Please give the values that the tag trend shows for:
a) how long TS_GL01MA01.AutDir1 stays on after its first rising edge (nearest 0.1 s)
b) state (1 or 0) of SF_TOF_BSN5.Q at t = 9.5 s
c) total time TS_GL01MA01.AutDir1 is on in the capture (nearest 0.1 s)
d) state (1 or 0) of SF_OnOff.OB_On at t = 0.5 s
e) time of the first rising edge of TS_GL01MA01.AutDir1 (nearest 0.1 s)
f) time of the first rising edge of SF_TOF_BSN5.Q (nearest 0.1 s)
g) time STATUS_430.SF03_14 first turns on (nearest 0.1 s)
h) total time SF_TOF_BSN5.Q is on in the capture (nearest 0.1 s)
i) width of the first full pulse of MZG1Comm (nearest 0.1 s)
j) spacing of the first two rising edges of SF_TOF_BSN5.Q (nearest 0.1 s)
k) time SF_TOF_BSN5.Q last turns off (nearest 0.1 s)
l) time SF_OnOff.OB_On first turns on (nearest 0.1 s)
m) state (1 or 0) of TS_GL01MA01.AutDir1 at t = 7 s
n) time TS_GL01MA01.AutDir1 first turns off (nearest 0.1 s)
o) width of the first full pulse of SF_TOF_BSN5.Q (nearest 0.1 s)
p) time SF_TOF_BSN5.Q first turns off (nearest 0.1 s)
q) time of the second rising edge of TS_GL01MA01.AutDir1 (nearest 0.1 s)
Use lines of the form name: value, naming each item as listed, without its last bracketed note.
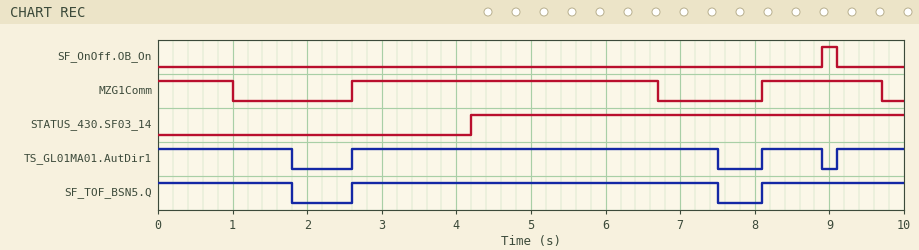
how long TS_GL01MA01.AutDir1 stays on after its first rising edge: 4.9 s
state (1 or 0) of SF_TOF_BSN5.Q at t = 9.5 s: 1
total time TS_GL01MA01.AutDir1 is on in the capture: 8.4 s
state (1 or 0) of SF_OnOff.OB_On at t = 0.5 s: 0
time of the first rising edge of TS_GL01MA01.AutDir1: 2.6 s
time of the first rising edge of SF_TOF_BSN5.Q: 2.6 s
time STATUS_430.SF03_14 first turns on: 4.2 s
total time SF_TOF_BSN5.Q is on in the capture: 8.6 s
width of the first full pulse of MZG1Comm: 4.1 s
spacing of the first two rising edges of SF_TOF_BSN5.Q: 5.5 s
time SF_TOF_BSN5.Q last turns off: 7.5 s
time SF_OnOff.OB_On first turns on: 8.9 s
state (1 or 0) of TS_GL01MA01.AutDir1 at t = 7 s: 1
time TS_GL01MA01.AutDir1 first turns off: 1.8 s
width of the first full pulse of SF_TOF_BSN5.Q: 4.9 s
time SF_TOF_BSN5.Q first turns off: 1.8 s
time of the second rising edge of TS_GL01MA01.AutDir1: 8.1 s
